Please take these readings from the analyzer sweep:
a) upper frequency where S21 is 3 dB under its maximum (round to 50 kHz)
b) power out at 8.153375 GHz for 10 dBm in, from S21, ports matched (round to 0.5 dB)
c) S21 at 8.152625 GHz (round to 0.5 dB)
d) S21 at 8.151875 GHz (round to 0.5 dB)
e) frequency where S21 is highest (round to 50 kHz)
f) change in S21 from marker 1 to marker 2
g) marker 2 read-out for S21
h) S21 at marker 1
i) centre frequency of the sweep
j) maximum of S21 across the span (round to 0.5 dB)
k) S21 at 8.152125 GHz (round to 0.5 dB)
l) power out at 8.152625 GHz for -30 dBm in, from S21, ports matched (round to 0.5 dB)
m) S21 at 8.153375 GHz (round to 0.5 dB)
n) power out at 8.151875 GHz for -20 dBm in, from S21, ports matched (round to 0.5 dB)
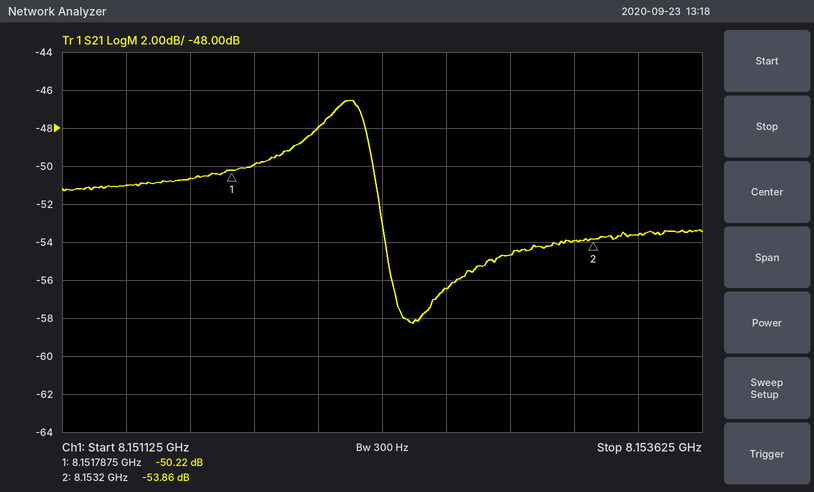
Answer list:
8.15235 GHz
-43.5 dBm
-56.5 dB
-50.0 dB
8.15225 GHz
-3.64 dB
-53.86 dB
-50.22 dB
8.152375 GHz
-46.5 dB
-48.0 dB
-86.5 dBm
-53.5 dB
-70.0 dBm
